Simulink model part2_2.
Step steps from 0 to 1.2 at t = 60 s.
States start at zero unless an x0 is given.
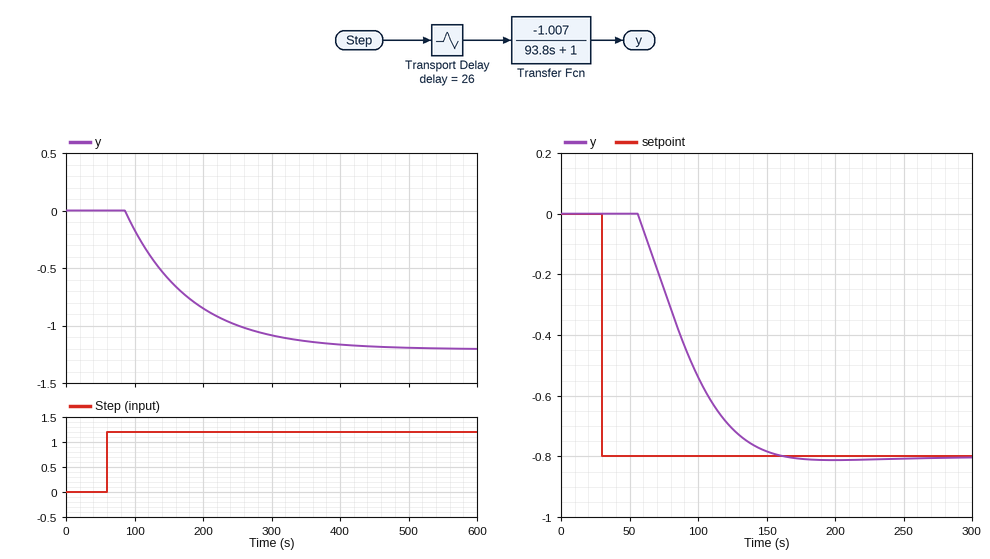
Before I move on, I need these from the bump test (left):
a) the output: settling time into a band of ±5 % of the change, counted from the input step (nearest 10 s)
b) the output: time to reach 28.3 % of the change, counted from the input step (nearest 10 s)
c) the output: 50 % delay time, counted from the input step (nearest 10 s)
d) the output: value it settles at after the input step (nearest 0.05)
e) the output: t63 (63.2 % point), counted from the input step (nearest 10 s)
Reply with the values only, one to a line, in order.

310 s
60 s
90 s
-1.20
120 s
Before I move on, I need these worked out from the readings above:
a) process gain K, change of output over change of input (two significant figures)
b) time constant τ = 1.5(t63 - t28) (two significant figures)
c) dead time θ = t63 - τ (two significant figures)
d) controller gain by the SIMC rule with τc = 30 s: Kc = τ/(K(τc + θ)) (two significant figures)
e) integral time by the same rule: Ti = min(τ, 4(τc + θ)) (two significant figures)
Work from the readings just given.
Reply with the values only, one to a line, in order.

-1.0
90 s
30 s
-1.5
90 s
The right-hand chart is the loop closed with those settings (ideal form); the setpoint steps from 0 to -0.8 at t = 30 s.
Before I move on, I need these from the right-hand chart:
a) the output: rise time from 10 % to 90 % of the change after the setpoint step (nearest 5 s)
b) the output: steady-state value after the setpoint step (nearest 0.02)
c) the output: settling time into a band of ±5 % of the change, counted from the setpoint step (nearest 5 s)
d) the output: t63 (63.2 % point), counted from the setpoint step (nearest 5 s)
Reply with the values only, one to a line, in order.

65 s
-0.80
110 s
65 s
